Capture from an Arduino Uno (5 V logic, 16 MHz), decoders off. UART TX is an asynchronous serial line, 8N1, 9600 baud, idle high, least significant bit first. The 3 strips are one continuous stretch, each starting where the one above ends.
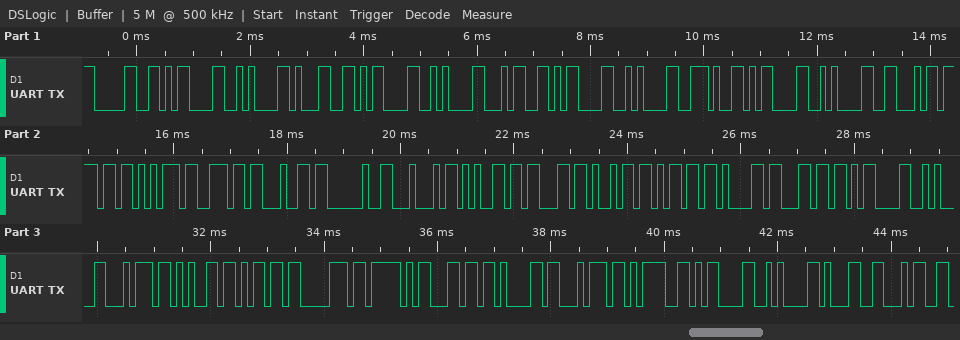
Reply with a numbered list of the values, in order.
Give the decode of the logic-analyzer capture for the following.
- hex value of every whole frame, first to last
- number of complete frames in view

1. 30 0D 0A 31 0D 0A 34 0D 0A 2E 0D 0A 46 6F 75 6E 64 20 44 65 63 69 6D 61 6C 0D 0A 74 65 6D 70 5F 6C 61 74 3D 0D 0A 31 34
2. 40
